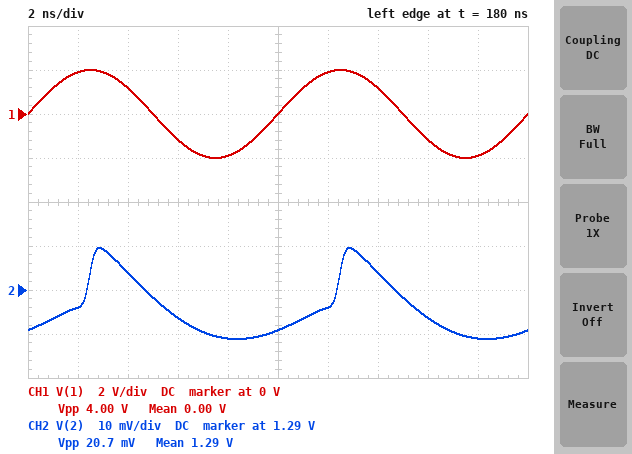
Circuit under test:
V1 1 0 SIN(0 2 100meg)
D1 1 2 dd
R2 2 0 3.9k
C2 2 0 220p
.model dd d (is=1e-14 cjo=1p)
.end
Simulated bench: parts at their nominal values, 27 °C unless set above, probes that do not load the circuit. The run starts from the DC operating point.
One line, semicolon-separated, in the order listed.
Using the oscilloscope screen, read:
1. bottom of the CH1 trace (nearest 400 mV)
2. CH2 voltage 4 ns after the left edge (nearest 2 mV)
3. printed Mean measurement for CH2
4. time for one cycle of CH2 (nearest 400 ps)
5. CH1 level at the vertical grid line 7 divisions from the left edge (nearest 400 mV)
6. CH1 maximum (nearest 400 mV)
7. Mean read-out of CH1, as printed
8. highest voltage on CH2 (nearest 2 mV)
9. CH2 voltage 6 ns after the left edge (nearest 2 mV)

-2.0 V; 1.294 V; 1.29 V; 10.0 ns; 1.2 V; 2.0 V; 0.00 V; 1.300 V; 1.284 V
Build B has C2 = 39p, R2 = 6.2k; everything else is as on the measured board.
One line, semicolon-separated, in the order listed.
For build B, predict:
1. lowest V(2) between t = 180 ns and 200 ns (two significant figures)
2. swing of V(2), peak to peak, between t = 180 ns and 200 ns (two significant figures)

1.2 V; 99 mV
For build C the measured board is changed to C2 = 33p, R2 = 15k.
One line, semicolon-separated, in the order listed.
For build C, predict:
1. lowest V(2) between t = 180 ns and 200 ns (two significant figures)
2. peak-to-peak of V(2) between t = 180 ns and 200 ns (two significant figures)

1.2 V; 99 mV
